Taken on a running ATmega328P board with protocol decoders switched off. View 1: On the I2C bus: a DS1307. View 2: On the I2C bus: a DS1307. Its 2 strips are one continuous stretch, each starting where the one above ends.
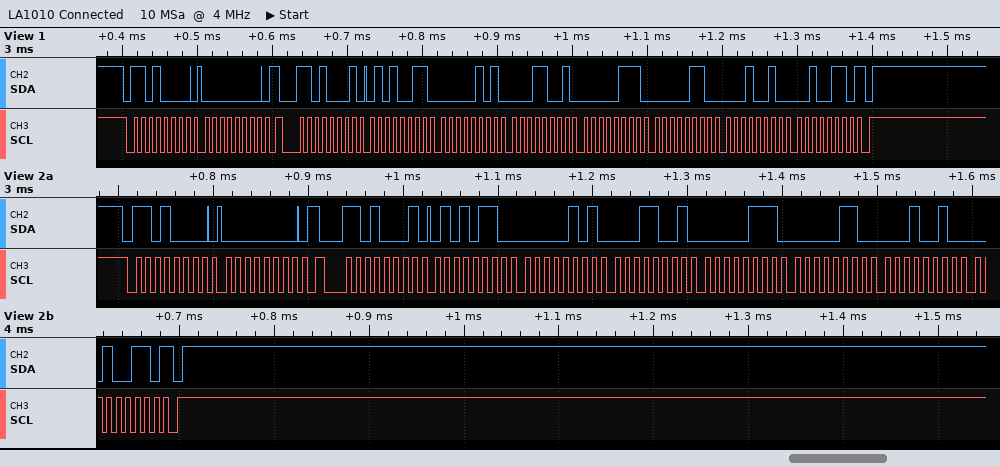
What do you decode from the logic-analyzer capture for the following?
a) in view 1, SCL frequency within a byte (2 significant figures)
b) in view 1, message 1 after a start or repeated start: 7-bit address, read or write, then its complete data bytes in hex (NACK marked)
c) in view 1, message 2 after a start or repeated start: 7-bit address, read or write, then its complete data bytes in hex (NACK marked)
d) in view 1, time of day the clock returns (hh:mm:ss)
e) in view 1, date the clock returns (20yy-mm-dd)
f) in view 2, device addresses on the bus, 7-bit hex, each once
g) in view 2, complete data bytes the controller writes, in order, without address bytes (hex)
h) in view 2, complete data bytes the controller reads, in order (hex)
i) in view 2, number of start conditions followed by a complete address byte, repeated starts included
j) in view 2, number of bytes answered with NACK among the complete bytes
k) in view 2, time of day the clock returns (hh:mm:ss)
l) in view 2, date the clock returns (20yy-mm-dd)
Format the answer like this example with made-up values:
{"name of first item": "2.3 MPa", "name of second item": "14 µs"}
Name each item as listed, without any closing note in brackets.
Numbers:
{"in view 1, SCL frequency within a byte": "100 kHz", "in view 1, message 1 after a start or repeated start: 7-bit address, read or write, then its complete data bytes in hex": "0x68 write: 00", "in view 1, message 2 after a start or repeated start: 7-bit address, read or write, then its complete data bytes in hex": "0x68 read: 53 05 19 07 06 12 26 NACK", "in view 1, time of day the clock returns": "19:05:53", "in view 1, date the clock returns": "2026-12-06", "in view 2, device addresses on the bus, 7-bit hex, each once": "0x68", "in view 2, complete data bytes the controller writes, in order, without address bytes": "00", "in view 2, complete data bytes the controller reads, in order": "56 05 19 07 06 12 26", "in view 2, number of start conditions followed by a complete address byte, repeated starts included": "2", "in view 2, number of bytes answered with NACK among the complete bytes": "1", "in view 2, time of day the clock returns": "19:05:56", "in view 2, date the clock returns": "2026-12-06"}
